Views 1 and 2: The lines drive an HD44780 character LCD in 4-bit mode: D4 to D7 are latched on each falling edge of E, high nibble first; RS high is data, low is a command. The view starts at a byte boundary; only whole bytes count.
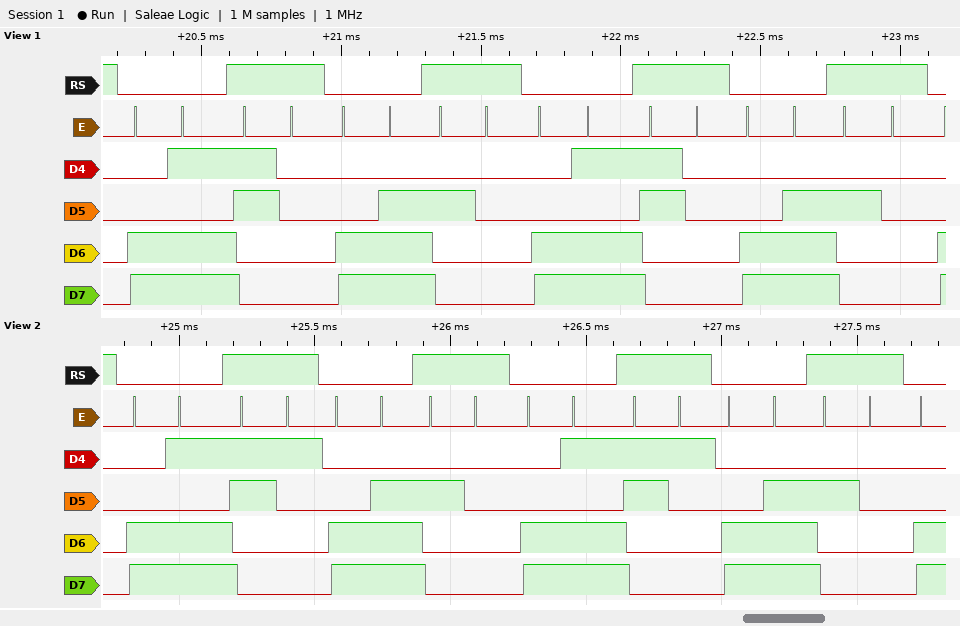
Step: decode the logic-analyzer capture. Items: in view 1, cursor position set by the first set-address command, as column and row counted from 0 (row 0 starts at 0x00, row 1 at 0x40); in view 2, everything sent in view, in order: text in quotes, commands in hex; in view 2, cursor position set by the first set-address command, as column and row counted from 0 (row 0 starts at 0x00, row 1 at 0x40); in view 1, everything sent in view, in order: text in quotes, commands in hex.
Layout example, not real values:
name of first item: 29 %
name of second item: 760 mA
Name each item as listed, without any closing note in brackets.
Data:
in view 1, cursor position set by the first set-address command, as column and row counted from 0: column 13, row 1
in view 2, everything sent in view, in order: text in quotes, commands in hex: 0xCD "1" 0xCE " " 0xCD "1" 0xCE " "
in view 2, cursor position set by the first set-address command, as column and row counted from 0: column 13, row 1
in view 1, everything sent in view, in order: text in quotes, commands in hex: 0xCD "0" 0xCE " " 0xCD "0" 0xCE " "
